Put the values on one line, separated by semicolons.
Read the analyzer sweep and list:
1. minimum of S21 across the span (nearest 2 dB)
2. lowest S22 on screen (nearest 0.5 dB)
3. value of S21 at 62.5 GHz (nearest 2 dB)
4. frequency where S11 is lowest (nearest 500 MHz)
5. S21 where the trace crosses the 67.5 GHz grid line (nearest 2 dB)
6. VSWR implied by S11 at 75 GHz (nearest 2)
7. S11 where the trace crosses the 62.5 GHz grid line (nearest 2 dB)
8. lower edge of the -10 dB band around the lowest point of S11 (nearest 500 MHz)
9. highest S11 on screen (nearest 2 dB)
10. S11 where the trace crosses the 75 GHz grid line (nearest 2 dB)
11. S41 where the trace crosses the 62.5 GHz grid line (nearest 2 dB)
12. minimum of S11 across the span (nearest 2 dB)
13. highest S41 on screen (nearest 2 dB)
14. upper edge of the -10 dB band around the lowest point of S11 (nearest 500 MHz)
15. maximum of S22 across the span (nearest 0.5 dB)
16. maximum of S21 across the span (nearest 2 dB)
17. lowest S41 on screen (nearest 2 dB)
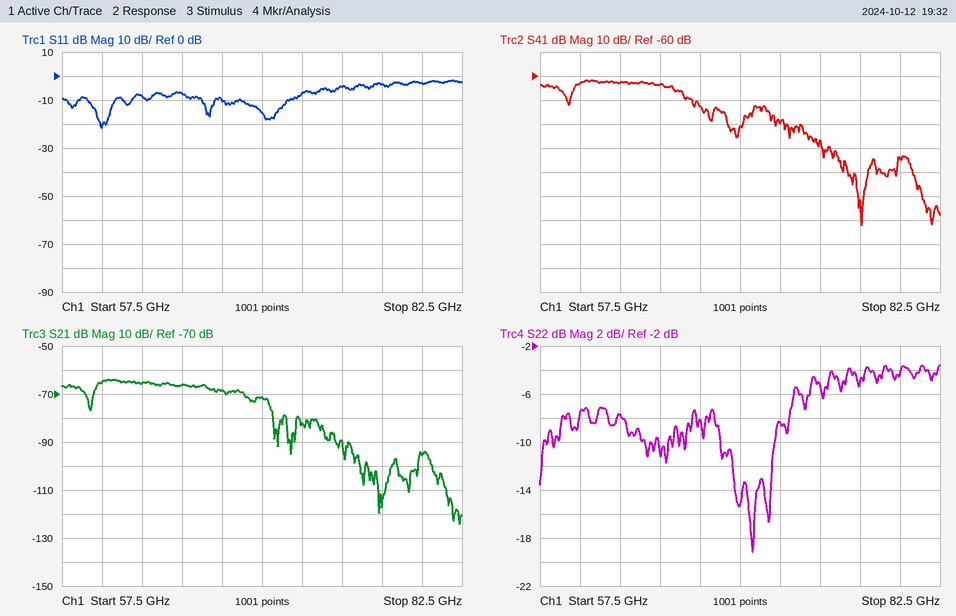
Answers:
-124 dB; -19.0 dB; -66 dB; 60.0 GHz; -68 dB; 4; -8 dB; 59.0 GHz; -2 dB; -4 dB; -62 dB; -22 dB; -62 dB; 61.0 GHz; -3.5 dB; -64 dB; -122 dB
